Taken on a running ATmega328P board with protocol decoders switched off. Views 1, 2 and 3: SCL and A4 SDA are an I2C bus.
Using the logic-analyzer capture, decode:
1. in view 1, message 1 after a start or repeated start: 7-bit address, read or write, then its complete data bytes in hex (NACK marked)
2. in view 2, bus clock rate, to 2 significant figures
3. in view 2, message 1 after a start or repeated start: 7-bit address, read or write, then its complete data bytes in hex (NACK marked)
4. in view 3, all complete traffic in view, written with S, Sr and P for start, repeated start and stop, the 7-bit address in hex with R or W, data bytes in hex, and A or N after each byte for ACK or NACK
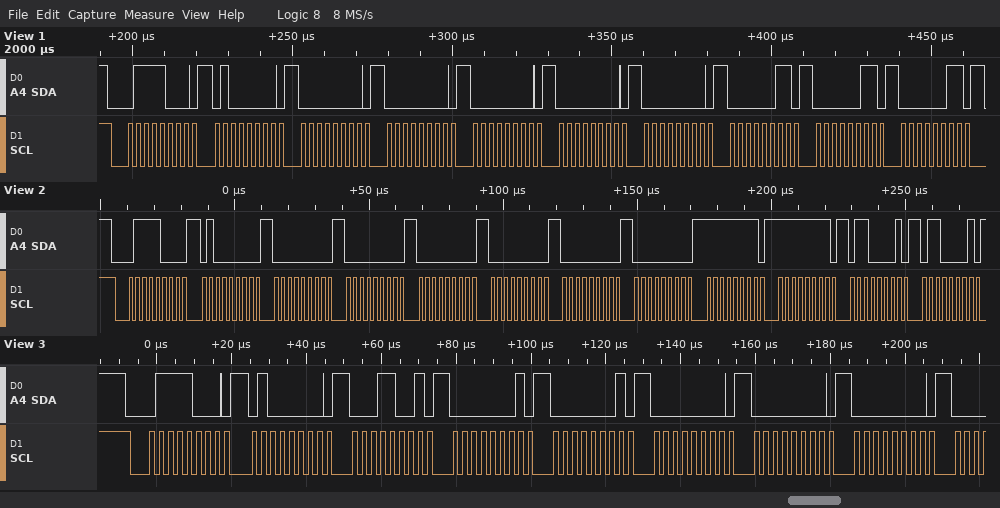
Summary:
0x3C write: 40 00 00 00 00 00 03 03 03
400 kHz
0x3C write: 40 00 00 00 00 00 00 FF FF 61 61
S 3CW A 40 A 19 A 01 A 01 A 00 A 00 A 00 A
